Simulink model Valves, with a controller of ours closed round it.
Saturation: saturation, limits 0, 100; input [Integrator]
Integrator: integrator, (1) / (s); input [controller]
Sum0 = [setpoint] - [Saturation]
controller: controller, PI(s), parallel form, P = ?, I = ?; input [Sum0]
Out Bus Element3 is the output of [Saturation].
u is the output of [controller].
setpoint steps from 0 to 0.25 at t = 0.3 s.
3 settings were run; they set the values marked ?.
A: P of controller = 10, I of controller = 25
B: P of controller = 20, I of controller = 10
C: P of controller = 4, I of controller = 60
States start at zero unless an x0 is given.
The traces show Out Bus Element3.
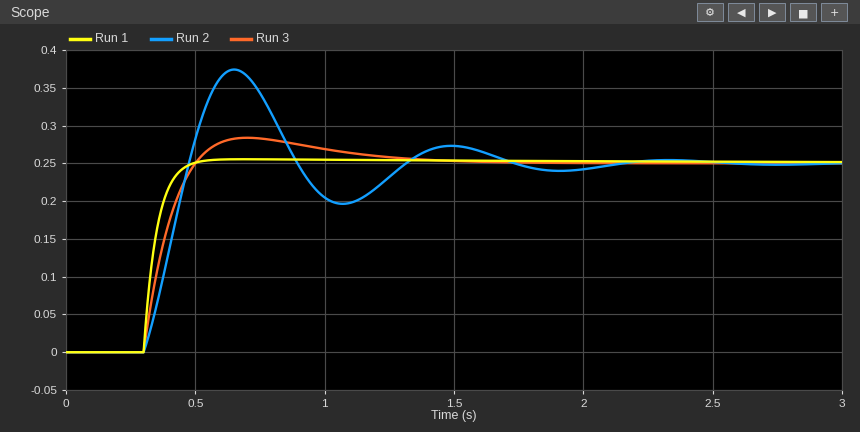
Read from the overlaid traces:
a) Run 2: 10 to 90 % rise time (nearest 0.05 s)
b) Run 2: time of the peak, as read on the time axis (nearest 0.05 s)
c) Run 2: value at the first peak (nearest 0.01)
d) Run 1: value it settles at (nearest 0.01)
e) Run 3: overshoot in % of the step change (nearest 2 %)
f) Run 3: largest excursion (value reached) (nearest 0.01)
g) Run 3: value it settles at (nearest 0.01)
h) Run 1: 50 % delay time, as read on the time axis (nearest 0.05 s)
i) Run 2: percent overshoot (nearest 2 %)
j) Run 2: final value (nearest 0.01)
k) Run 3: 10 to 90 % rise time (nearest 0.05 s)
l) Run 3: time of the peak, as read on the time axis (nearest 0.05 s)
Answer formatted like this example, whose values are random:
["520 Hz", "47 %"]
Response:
["0.15 s", "0.65 s", "0.37", "0.25", "14 %", "0.28", "0.25", "0.35 s", "50 %", "0.25", "0.15 s", "0.70 s"]
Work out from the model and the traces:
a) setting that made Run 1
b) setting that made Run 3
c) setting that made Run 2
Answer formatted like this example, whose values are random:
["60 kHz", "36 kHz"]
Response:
["B", "A", "C"]
